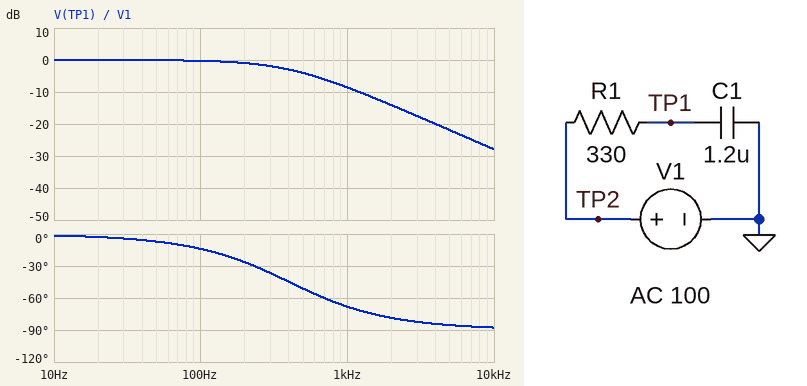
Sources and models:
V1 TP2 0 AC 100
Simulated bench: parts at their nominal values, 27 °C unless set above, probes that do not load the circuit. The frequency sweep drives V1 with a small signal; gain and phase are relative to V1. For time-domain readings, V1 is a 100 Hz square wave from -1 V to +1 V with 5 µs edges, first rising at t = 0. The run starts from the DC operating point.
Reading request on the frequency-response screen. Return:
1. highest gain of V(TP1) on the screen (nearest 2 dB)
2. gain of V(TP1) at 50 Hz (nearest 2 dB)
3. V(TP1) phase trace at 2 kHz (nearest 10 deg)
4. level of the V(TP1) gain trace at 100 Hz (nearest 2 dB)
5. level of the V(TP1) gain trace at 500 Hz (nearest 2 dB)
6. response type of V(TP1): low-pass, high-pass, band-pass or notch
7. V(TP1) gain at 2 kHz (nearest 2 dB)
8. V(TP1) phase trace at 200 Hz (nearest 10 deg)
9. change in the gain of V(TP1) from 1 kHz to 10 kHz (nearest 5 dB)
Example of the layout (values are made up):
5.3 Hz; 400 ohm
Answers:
0 dB; 0 dB; -80 deg; 0 dB; -4 dB; low-pass; -14 dB; -30 deg; -20 dB
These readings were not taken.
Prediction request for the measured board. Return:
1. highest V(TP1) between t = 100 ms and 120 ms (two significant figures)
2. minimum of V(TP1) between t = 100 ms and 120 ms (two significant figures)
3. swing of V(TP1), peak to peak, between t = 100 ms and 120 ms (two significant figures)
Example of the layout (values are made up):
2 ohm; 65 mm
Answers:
1.0 V; -1.0 V; 2.0 V
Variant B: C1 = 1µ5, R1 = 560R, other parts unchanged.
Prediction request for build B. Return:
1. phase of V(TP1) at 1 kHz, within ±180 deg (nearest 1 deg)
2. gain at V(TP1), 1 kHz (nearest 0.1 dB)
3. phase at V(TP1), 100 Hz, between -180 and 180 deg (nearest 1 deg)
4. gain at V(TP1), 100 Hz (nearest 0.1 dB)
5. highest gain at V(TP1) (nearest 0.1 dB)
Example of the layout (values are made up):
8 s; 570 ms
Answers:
-79 deg; -14.6 dB; -28 deg; -1.1 dB; 0 dB
